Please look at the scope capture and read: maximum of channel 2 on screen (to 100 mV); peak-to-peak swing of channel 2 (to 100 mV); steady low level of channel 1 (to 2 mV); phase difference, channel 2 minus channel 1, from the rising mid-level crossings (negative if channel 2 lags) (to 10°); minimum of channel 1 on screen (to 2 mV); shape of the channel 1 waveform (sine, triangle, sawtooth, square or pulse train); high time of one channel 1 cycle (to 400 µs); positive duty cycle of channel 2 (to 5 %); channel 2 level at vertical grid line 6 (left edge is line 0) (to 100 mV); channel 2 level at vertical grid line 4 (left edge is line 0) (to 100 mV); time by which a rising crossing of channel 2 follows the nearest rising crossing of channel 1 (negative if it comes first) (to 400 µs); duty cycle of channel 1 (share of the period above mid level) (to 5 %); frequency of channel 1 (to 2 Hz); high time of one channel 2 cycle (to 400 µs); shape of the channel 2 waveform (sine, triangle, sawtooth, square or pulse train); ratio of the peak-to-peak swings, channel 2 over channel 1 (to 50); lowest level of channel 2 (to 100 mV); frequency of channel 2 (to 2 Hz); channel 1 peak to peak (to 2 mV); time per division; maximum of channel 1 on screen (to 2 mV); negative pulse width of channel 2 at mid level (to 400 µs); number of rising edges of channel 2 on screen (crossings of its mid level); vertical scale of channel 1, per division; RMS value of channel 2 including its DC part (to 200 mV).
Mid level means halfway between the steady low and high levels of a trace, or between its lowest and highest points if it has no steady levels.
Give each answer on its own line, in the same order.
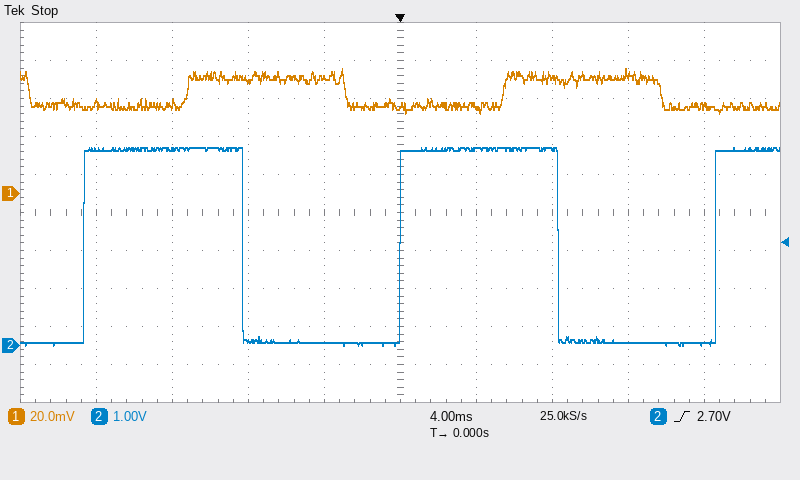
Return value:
5.2 V
5.2 V
46 mV
+120°
42 mV
square
8.4 ms
50 %
5.2 V
100 mV
-5.6 ms
50 %
60 Hz
8.4 ms
square
200
0.0 V
60 Hz
24 mV
4 ms
66 mV
8.4 ms
3
20 mV
3.6 V
